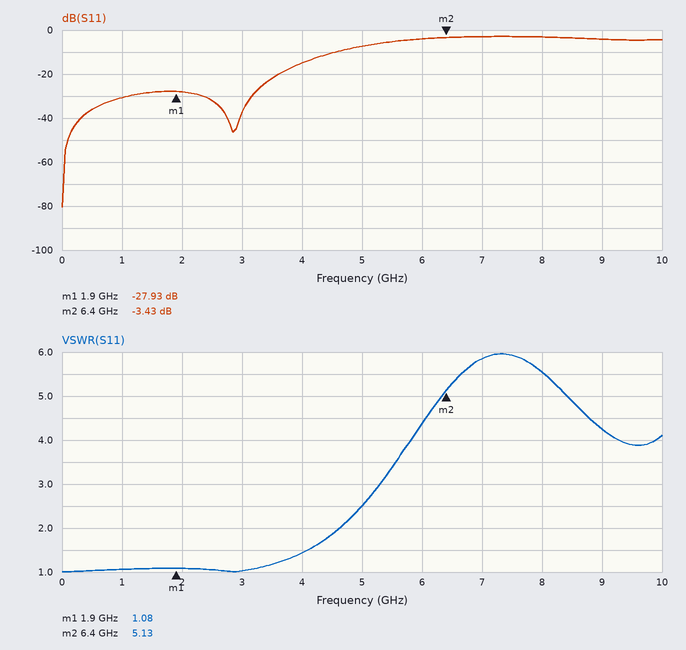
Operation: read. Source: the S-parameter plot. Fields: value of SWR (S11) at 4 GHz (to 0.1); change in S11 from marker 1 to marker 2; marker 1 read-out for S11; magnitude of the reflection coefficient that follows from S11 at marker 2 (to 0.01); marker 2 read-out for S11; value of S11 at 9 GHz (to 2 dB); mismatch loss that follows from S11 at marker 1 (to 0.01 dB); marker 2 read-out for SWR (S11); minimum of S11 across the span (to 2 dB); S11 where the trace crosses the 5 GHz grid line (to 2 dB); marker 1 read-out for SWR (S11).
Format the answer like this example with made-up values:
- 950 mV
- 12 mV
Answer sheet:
- 1.4
- 24.50 dB
- -27.93 dB
- 0.67
- -3.43 dB
- -4 dB
- 0.01 dB
- 5.13
- -80 dB
- -8 dB
- 1.08
